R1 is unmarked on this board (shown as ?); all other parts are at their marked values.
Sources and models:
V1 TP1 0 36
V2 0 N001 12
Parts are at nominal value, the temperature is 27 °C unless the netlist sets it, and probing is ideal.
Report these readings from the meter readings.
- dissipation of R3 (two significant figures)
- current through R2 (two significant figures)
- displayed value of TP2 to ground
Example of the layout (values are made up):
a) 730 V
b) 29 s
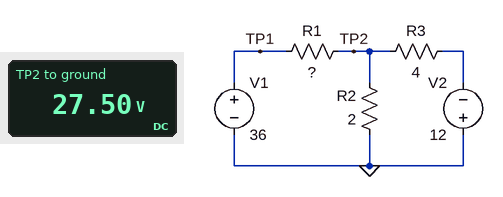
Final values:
a) 390 W
b) 14 A
c) 27.50 V
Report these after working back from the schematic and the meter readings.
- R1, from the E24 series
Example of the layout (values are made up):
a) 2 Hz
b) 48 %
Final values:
a) 0.36 Ω
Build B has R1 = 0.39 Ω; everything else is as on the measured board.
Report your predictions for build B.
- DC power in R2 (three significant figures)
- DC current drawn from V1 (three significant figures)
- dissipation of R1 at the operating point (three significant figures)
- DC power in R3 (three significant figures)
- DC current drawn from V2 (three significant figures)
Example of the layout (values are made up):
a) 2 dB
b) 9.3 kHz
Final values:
a) 363 W
b) 23.2 A
c) 210 W
d) 379 W
e) 9.74 A
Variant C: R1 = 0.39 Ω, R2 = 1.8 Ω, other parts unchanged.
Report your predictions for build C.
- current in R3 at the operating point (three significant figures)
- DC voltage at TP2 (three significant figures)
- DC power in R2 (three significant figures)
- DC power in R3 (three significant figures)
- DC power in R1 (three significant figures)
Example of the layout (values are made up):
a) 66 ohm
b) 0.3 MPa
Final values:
a) 9.63 A
b) 26.5 V
c) 390 W
d) 371 W
e) 231 W
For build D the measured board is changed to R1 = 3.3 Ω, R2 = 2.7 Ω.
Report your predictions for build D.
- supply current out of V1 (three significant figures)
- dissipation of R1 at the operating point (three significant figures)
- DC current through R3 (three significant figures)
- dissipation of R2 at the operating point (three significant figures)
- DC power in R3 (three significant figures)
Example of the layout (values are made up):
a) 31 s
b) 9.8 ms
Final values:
a) 8.31 A
b) 228 W
c) 5.14 A
d) 27.2 W
e) 106 W
